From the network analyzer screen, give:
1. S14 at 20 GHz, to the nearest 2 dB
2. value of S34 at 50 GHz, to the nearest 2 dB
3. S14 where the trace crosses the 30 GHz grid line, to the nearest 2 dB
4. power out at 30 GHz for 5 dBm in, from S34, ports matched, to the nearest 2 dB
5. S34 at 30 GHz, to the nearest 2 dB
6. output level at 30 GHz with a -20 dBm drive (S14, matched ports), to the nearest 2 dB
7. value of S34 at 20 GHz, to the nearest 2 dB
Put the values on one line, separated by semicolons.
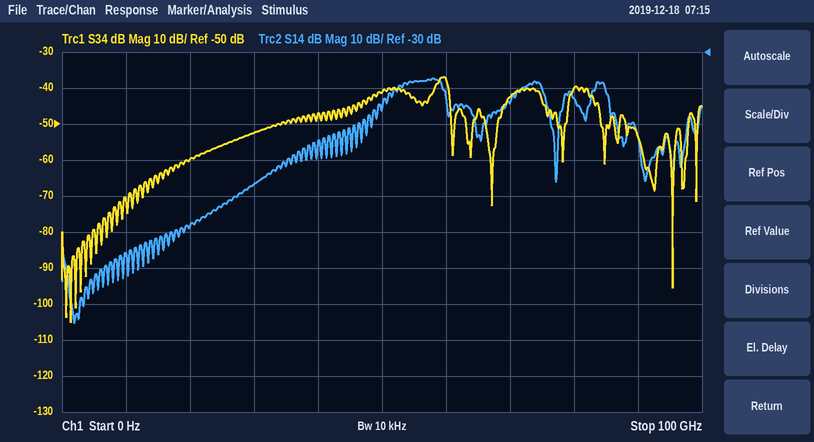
-78 dB; -42 dB; -66 dB; -48 dBm; -52 dB; -86 dBm; -60 dB
